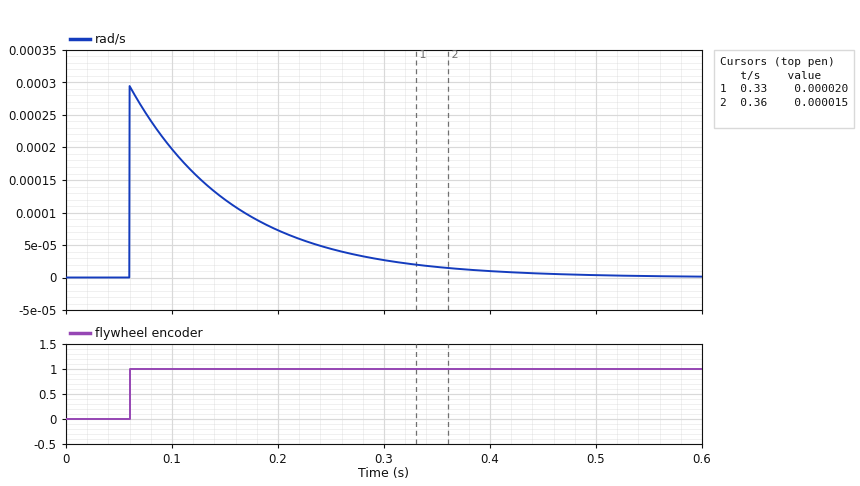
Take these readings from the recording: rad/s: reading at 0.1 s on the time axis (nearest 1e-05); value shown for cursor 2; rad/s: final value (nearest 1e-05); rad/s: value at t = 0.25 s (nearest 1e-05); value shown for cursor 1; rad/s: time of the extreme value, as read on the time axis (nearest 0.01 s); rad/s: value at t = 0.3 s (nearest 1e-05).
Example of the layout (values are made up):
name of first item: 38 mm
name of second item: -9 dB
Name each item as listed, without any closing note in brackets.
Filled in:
rad/s: reading at 0.1 s on the time axis: 0.00020
value shown for cursor 2: 0.000015
rad/s: final value: 0.00000
rad/s: value at t = 0.25 s: 0.00004
value shown for cursor 1: 0.000020
rad/s: time of the extreme value, as read on the time axis: 0.06 s
rad/s: value at t = 0.3 s: 0.00003
